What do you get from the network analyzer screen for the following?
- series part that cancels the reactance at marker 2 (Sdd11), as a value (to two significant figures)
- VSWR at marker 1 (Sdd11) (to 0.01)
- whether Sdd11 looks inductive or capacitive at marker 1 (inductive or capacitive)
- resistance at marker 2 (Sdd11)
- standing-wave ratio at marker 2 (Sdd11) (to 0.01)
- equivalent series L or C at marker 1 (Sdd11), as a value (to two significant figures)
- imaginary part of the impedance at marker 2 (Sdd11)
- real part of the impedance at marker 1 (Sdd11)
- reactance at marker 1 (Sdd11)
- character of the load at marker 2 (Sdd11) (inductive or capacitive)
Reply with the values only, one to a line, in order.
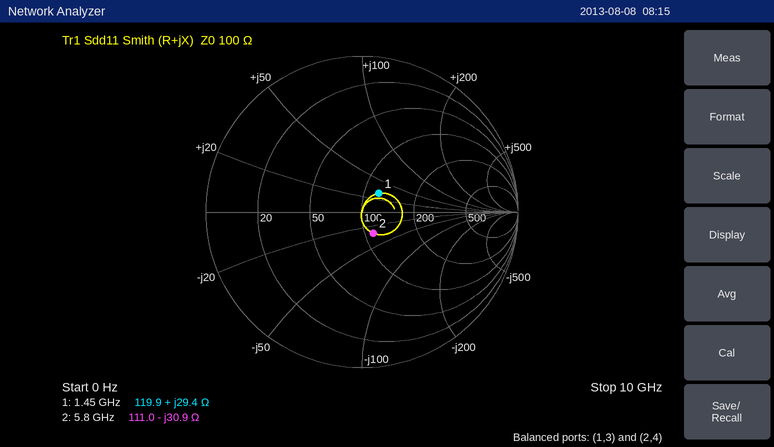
850 pH
1.38
inductive
111.0 Ω
1.36
3.2 nH
-30.9 Ω
119.9 Ω
+29.4 Ω
capacitive
